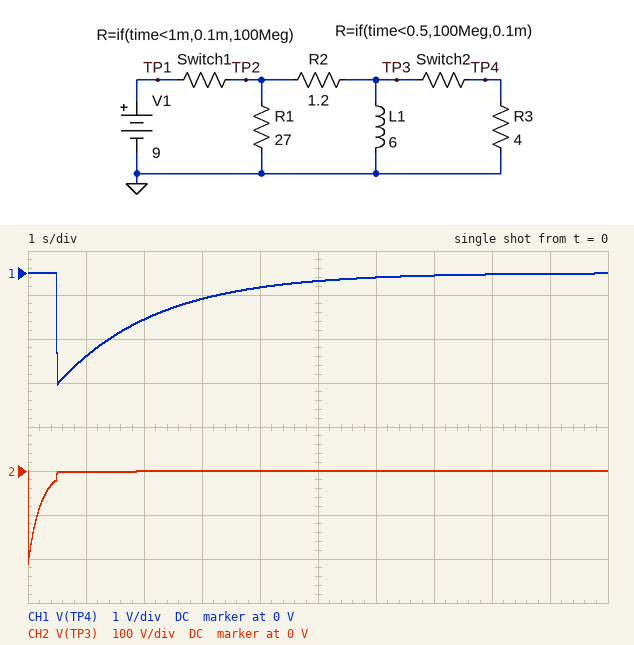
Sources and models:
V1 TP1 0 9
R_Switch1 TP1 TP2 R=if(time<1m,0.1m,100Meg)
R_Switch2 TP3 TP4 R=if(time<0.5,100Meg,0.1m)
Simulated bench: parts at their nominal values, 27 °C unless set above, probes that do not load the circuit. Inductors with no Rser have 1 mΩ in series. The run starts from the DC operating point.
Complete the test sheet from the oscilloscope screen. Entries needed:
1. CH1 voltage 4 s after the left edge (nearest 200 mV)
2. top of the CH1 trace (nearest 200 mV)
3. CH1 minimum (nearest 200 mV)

-400 mV
0 V
-2.6 V
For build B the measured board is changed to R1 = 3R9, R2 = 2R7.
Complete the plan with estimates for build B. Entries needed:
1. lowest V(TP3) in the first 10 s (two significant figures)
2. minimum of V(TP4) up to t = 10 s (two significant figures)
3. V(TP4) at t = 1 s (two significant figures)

-22 V
-4.8 V
-3.9 V
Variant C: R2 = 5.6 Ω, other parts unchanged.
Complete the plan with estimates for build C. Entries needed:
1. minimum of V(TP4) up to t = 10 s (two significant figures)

-380 mV
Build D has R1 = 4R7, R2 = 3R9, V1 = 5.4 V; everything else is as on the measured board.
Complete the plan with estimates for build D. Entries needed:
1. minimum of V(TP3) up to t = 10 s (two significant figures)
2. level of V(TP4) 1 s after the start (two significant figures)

-12 V
-1.5 V
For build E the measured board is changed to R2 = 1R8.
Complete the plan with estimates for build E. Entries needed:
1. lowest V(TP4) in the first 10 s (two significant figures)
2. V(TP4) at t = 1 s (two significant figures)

-1.6 V
-1.2 V
